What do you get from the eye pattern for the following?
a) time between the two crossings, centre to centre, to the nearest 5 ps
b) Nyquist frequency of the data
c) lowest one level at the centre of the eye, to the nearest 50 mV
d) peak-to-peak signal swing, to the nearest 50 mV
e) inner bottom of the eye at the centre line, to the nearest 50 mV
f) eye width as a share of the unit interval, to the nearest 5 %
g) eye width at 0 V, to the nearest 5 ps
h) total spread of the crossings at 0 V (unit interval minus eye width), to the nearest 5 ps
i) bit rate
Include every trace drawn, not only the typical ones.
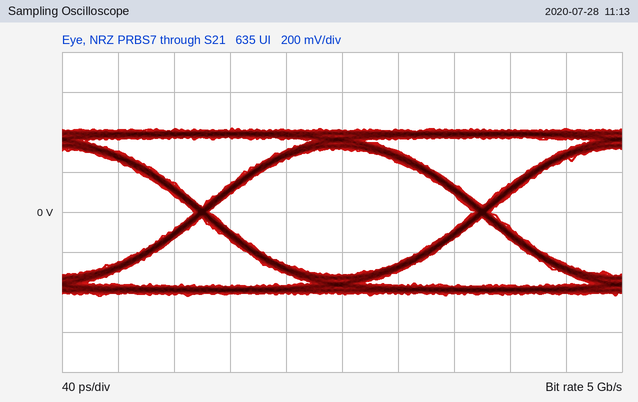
200 ps
2.5 GHz
300 mV
850 mV
-300 mV
95 %
190 ps
10 ps
5 Gb/s
